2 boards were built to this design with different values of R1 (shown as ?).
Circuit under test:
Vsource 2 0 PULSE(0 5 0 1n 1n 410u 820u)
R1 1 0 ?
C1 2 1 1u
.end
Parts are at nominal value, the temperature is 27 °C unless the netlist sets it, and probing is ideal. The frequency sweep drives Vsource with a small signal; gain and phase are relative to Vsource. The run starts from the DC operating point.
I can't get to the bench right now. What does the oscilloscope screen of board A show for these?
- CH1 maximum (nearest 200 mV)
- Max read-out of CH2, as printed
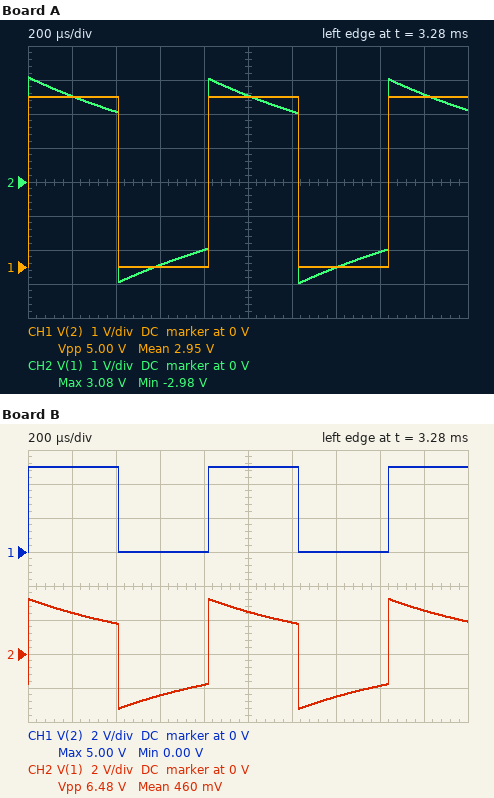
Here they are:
5.0 V
3.08 V
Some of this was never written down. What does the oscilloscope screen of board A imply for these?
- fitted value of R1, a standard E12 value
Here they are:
1 kΩ
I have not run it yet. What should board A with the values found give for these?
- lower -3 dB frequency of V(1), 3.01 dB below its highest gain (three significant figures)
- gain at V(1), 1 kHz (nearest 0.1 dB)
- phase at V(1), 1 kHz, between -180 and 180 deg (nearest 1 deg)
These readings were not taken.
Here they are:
159 Hz
-0.1 dB
9 deg
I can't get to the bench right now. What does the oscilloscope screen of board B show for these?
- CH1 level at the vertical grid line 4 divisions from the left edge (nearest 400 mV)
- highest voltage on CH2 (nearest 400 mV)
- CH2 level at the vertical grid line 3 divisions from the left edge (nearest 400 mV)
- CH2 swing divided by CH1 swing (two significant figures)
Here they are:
0 V
3.2 V
-2.4 V
1.3
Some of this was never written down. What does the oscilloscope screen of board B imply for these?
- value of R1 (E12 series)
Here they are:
680 Ω
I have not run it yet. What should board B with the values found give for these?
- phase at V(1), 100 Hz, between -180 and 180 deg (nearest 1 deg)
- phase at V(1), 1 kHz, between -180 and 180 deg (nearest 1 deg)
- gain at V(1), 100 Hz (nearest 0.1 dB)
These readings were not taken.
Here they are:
67 deg
13 deg
-8.1 dB
